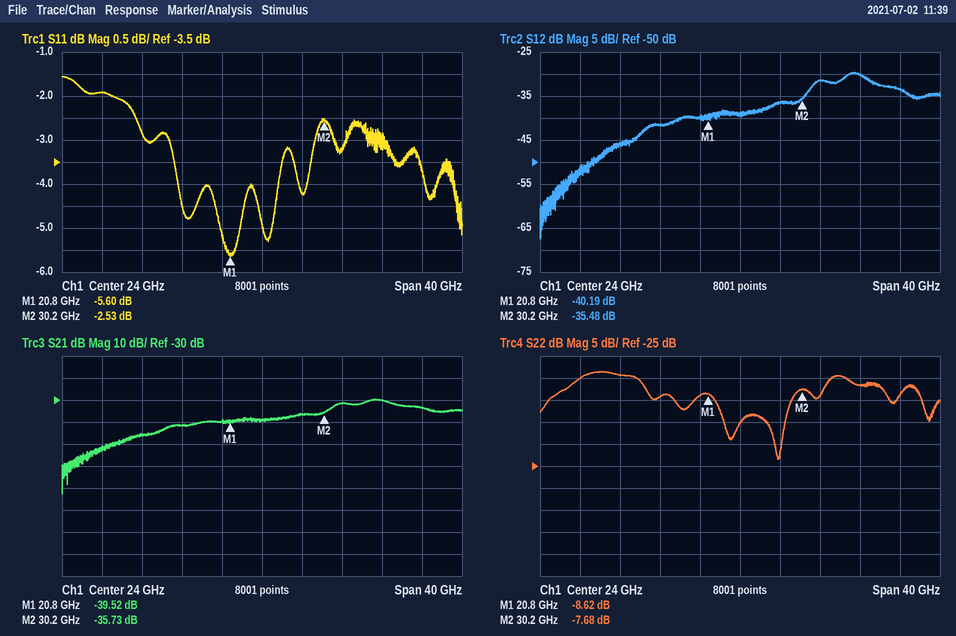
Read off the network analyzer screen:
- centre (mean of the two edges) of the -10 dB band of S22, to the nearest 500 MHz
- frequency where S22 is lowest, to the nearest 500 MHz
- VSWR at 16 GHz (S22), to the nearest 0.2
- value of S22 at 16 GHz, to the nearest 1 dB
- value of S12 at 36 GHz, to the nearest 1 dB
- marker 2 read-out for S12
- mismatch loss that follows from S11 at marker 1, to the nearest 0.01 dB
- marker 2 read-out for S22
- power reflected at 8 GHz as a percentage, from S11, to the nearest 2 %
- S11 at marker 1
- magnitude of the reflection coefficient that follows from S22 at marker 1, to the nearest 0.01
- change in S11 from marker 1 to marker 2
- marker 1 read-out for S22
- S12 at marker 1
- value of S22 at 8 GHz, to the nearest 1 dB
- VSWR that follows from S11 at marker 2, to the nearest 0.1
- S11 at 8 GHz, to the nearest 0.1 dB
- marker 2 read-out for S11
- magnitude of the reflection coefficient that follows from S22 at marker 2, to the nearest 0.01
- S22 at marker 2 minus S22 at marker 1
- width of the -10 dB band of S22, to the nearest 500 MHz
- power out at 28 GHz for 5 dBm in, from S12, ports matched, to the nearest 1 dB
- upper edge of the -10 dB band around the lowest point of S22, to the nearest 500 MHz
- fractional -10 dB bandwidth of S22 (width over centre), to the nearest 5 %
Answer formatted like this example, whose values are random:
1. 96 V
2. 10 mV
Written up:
1. 25.5 GHz
2. 28.0 GHz
3. 2.0
4. -9 dB
5. -30 dB
6. -35.48 dB
7. 1.40 dB
8. -7.68 dB
9. 64 %
10. -5.60 dB
11. 0.37
12. 3.07 dB
13. -8.62 dB
14. -40.19 dB
15. -5 dB
16. 6.9
17. -1.9 dB
18. -2.53 dB
19. 0.41
20. 0.94 dB
21. 7.5 GHz
22. -31 dBm
23. 29.0 GHz
24. 30 %
